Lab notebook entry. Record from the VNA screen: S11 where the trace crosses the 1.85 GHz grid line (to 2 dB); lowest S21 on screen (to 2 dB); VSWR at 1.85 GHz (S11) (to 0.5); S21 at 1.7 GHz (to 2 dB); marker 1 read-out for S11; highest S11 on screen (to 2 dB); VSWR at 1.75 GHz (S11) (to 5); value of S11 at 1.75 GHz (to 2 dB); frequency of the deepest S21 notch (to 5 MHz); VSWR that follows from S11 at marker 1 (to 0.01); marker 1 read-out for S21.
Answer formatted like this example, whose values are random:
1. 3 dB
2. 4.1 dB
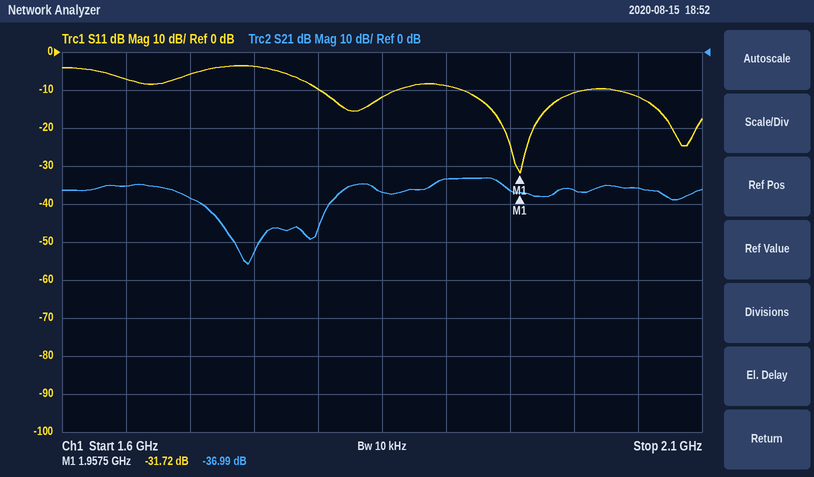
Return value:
1. -12 dB
2. -56 dB
3. 1.5
4. -38 dB
5. -31.72 dB
6. -4 dB
7. 5
8. -4 dB
9. 1.745 GHz
10. 1.05
11. -36.99 dB
